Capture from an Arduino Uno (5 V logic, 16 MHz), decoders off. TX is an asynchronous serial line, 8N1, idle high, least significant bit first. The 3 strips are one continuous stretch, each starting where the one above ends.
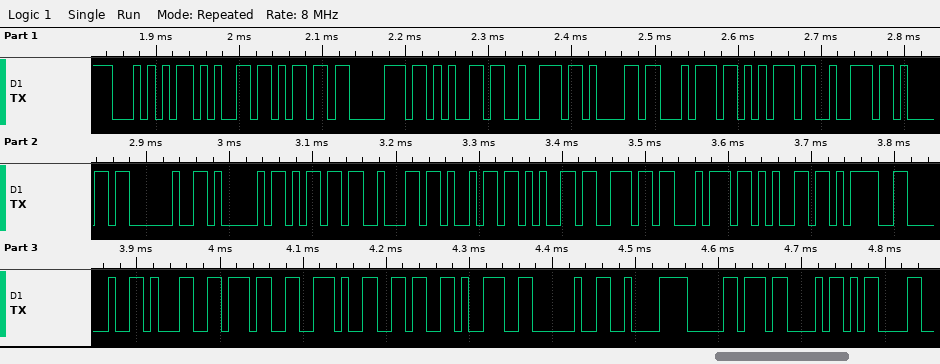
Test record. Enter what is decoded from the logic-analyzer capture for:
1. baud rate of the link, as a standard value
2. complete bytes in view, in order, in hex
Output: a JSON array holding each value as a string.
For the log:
["115200 baud", "54 65 6D 70 65 72 61 74 75 72 61 20 41 6D 62 69 65 6E 74 65 3D 20 31 37 2E 36 39 20 C2 B0 43 0D"]
